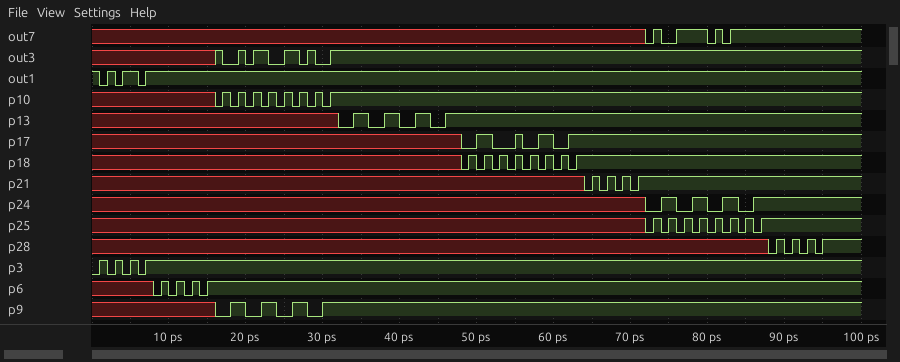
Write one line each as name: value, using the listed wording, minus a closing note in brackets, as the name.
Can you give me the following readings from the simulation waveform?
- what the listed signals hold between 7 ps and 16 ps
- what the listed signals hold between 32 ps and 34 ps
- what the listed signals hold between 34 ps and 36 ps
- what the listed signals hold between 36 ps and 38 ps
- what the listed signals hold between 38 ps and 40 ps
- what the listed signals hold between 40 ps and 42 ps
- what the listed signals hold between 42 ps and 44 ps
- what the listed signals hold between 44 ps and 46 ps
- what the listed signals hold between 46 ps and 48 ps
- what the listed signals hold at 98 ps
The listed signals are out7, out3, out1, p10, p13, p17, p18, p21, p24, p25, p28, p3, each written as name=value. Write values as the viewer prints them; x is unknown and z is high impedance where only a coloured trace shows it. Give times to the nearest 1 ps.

what the listed signals hold between 7 ps and 16 ps: out7=x, out3=x, out1=1, p10=x, p13=x, p17=x, p18=x, p21=x, p24=x, p25=x, p28=x, p3=1
what the listed signals hold between 32 ps and 34 ps: out7=x, out3=1, out1=1, p10=1, p13=0, p17=x, p18=x, p21=x, p24=x, p25=x, p28=x, p3=1
what the listed signals hold between 34 ps and 36 ps: out7=x, out3=1, out1=1, p10=1, p13=1, p17=x, p18=x, p21=x, p24=x, p25=x, p28=x, p3=1
what the listed signals hold between 36 ps and 38 ps: out7=x, out3=1, out1=1, p10=1, p13=0, p17=x, p18=x, p21=x, p24=x, p25=x, p28=x, p3=1
what the listed signals hold between 38 ps and 40 ps: out7=x, out3=1, out1=1, p10=1, p13=1, p17=x, p18=x, p21=x, p24=x, p25=x, p28=x, p3=1
what the listed signals hold between 40 ps and 42 ps: out7=x, out3=1, out1=1, p10=1, p13=0, p17=x, p18=x, p21=x, p24=x, p25=x, p28=x, p3=1
what the listed signals hold between 42 ps and 44 ps: out7=x, out3=1, out1=1, p10=1, p13=1, p17=x, p18=x, p21=x, p24=x, p25=x, p28=x, p3=1
what the listed signals hold between 44 ps and 46 ps: out7=x, out3=1, out1=1, p10=1, p13=0, p17=x, p18=x, p21=x, p24=x, p25=x, p28=x, p3=1
what the listed signals hold between 46 ps and 48 ps: out7=x, out3=1, out1=1, p10=1, p13=1, p17=x, p18=x, p21=x, p24=x, p25=x, p28=x, p3=1
what the listed signals hold at 98 ps: out7=1, out3=1, out1=1, p10=1, p13=1, p17=1, p18=1, p21=1, p24=1, p25=1, p28=1, p3=1
